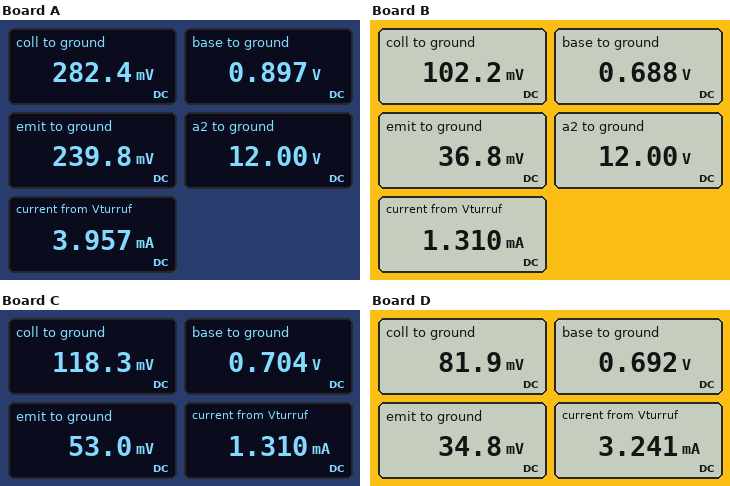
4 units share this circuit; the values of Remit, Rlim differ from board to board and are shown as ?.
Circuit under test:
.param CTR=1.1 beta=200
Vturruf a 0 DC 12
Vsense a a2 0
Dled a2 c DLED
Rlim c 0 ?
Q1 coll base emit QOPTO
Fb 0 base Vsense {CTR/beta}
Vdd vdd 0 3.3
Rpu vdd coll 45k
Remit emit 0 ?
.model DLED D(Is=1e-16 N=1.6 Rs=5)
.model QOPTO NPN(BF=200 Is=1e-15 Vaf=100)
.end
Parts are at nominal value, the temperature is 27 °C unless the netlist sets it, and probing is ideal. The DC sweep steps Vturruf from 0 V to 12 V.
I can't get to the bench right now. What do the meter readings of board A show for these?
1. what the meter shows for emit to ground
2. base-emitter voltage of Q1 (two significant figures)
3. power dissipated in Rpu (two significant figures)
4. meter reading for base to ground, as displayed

239.8 mV
660 mV
200 µW
0.897 V
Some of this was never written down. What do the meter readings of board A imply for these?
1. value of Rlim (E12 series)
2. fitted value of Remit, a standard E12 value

2.7 kΩ
2.7 kΩ
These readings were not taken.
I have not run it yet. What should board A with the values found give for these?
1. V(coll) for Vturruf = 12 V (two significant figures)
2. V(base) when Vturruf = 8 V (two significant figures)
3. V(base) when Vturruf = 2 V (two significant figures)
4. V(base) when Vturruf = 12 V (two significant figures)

280 mV
870 mV
830 mV
900 mV
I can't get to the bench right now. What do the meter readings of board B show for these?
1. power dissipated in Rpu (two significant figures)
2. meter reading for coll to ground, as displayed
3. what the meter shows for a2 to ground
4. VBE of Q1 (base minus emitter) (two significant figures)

230 µW
102.2 mV
12.00 V
650 mV
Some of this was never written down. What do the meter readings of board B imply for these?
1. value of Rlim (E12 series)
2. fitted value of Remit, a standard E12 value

8.2 kΩ
470 Ω
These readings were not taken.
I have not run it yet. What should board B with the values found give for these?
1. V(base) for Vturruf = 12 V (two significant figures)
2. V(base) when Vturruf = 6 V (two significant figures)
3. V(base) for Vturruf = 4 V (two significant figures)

690 mV
680 mV
680 mV
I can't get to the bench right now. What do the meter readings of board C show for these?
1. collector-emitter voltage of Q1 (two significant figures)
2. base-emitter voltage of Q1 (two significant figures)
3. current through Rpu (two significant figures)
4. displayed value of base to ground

65 mV
650 mV
71 µA
0.704 V
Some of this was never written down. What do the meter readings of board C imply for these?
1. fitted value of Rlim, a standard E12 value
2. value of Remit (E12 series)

8.2 kΩ
680 Ω
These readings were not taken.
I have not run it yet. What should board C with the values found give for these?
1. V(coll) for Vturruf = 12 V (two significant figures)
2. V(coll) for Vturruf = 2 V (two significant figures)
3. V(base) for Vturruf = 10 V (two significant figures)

120 mV
200 mV
700 mV
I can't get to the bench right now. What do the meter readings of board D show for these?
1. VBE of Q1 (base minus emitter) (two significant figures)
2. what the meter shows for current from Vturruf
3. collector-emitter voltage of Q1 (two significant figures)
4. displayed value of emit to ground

660 mV
3.241 mA
47 mV
34.8 mV
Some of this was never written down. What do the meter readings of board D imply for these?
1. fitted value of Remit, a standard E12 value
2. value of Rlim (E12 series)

390 Ω
3.3 kΩ
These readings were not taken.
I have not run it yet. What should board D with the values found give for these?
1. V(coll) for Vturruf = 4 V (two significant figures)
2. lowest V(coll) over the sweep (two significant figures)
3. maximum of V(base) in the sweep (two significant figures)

110 mV
82 mV
690 mV
